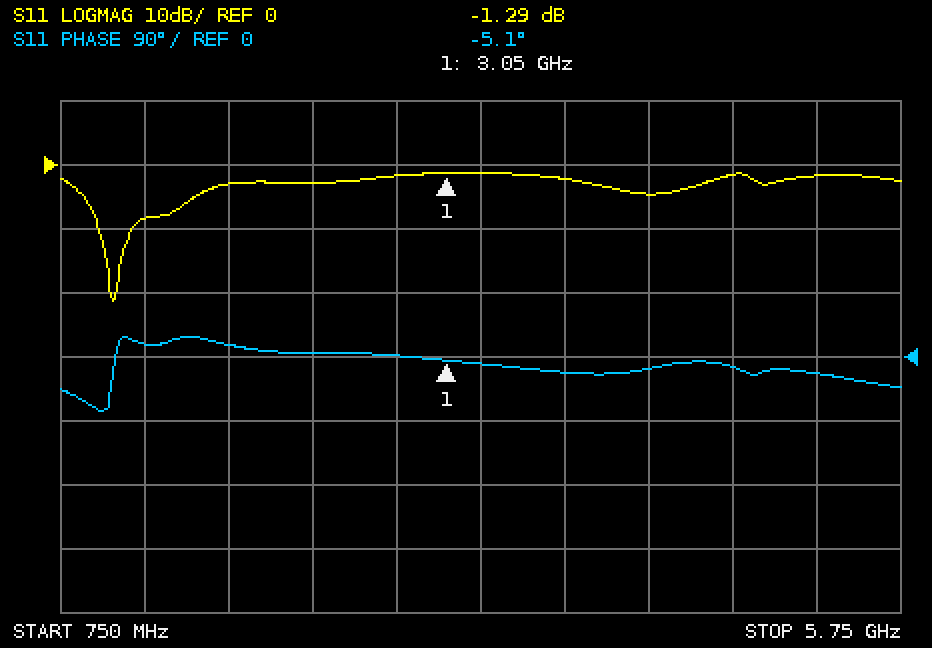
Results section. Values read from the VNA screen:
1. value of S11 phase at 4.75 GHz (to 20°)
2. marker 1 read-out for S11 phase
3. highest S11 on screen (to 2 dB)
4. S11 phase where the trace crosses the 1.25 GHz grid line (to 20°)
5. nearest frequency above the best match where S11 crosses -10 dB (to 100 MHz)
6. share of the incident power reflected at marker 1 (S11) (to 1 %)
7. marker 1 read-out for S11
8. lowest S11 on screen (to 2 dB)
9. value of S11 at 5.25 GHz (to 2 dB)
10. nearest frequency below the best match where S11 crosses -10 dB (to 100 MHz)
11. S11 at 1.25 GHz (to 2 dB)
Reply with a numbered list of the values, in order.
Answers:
1. -20°
2. -5.1°
3. -2 dB
4. 20°
5. 1.2 GHz
6. 74 %
7. -1.29 dB
8. -22 dB
9. -2 dB
10. 1.0 GHz
11. -8 dB
